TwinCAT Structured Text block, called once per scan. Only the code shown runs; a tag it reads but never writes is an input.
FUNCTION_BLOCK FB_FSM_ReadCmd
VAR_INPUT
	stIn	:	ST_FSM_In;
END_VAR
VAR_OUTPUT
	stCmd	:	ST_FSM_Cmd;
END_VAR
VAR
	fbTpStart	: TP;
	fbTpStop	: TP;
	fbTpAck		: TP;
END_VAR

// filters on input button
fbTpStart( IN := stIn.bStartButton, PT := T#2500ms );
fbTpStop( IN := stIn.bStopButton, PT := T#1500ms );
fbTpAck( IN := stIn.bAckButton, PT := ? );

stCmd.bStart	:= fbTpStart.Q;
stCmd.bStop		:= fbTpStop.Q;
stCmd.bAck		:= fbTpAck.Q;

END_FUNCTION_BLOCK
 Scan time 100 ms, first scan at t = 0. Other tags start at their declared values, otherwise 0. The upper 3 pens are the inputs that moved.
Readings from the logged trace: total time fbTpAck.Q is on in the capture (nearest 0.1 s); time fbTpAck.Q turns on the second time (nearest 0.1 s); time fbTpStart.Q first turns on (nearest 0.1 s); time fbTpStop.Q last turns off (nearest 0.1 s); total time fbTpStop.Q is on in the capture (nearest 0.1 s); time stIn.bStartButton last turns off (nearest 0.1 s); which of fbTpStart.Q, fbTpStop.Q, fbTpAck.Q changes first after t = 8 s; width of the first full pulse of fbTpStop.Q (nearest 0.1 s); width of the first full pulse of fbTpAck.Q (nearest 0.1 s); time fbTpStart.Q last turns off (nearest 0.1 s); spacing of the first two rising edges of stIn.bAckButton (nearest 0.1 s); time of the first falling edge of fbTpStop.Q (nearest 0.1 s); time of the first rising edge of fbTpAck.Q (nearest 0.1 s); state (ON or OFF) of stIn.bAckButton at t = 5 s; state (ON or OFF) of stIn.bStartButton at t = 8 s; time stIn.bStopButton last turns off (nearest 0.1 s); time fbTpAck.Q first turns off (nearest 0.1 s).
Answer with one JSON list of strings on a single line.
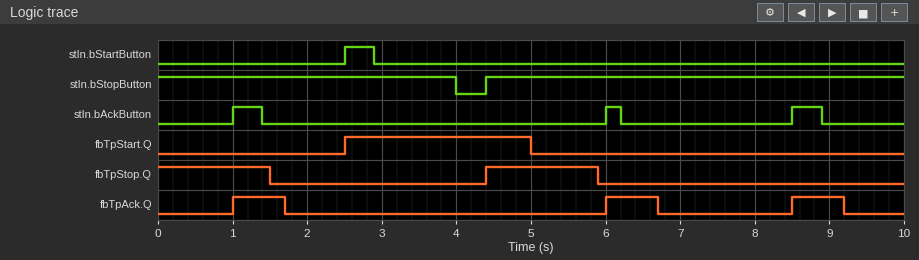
["2.1 s", "6.0 s", "2.5 s", "5.9 s", "3.0 s", "2.9 s", "fbTpAck.Q", "1.5 s", "0.7 s", "5.0 s", "5.0 s", "1.5 s", "1.0 s", "OFF", "OFF", "4.0 s", "1.7 s"]
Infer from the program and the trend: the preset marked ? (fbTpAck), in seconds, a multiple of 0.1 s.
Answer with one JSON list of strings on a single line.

["0.7 s"]
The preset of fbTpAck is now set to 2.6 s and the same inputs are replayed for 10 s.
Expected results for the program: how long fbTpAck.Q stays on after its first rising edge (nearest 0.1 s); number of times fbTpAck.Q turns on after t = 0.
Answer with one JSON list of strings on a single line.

["2.6 s", "2"]
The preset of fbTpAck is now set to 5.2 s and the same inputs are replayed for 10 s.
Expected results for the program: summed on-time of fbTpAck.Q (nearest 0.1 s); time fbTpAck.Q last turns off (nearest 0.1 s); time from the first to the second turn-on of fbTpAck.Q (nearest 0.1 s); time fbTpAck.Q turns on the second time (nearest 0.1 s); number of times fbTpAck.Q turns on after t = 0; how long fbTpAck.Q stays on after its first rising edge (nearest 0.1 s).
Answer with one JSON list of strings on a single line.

["6.7 s", "6.2 s", "7.5 s", "8.5 s", "2", "5.2 s"]
